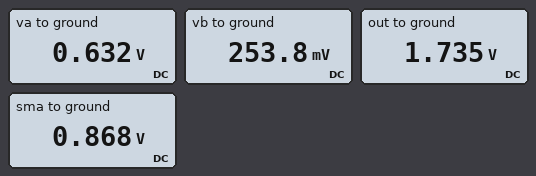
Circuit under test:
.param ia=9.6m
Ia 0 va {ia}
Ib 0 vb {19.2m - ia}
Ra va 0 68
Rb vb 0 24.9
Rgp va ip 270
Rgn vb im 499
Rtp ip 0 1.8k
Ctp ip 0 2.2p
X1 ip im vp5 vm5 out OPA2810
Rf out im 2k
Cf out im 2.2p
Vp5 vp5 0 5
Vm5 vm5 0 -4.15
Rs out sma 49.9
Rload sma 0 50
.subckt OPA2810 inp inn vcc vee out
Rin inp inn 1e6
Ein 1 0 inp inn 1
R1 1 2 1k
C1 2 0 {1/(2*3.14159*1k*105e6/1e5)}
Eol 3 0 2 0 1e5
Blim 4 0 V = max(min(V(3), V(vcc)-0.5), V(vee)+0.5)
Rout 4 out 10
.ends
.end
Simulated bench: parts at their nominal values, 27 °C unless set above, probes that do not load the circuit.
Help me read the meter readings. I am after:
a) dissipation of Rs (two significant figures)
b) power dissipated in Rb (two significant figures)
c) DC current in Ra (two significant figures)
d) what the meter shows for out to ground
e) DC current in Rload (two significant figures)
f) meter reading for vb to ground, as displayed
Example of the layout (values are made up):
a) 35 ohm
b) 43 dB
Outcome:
a) 15 mW
b) 2.6 mW
c) 9.3 mA
d) 1.735 V
e) 17 mA
f) 253.8 mV
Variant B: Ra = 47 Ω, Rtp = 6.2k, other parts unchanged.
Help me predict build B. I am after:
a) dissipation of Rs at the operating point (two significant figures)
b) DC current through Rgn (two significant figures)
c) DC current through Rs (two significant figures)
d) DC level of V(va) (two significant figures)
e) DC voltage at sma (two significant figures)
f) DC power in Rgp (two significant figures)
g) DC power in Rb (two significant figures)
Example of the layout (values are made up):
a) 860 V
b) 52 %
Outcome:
a) 6.7 mW
b) 360 µA
c) 12 mA
d) 450 mV
e) 580 mV
f) 1.3 µW
g) 2.5 mW
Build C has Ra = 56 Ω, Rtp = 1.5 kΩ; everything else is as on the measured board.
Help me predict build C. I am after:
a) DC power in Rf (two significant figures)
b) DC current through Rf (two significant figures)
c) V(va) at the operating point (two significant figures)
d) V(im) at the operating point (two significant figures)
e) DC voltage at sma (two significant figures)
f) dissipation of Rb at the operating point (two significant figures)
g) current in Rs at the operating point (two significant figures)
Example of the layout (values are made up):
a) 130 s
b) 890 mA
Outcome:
a) 300 µW
b) 390 µA
c) 520 mV
d) 440 mV
e) 610 mV
f) 2.5 mW
g) 12 mA
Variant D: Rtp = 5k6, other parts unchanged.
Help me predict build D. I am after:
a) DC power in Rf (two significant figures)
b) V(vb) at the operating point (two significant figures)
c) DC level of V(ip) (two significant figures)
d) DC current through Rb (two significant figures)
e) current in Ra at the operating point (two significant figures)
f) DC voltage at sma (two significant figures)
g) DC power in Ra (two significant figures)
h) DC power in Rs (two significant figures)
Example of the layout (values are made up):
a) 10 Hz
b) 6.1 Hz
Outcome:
a) 1.0 mW
b) 260 mV
c) 620 mV
d) 10 mA
e) 9.5 mA
f) 1.0 V
g) 6.1 mW
h) 21 mW
